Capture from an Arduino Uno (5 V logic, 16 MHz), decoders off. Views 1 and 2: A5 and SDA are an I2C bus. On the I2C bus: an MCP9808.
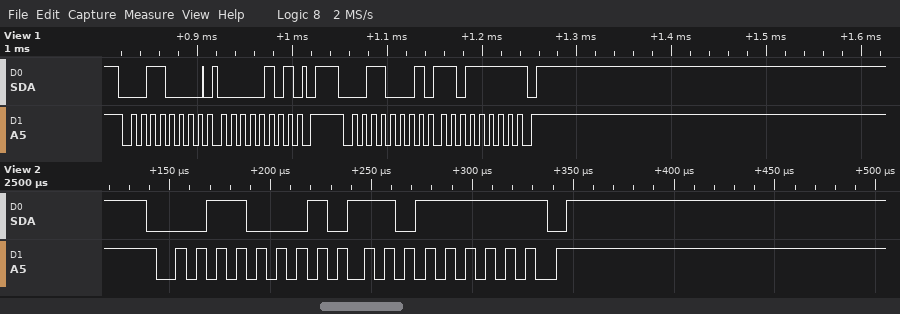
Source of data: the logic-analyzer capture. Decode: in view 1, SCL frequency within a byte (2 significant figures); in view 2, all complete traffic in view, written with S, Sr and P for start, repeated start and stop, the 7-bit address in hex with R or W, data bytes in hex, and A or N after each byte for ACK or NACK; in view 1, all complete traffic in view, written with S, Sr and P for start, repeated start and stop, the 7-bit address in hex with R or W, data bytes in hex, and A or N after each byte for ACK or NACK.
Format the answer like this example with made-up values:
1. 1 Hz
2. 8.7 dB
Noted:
1. 100 kHz
2. S 18R A DF N P
3. S 18W A 05 A P S 18R A DF N P
